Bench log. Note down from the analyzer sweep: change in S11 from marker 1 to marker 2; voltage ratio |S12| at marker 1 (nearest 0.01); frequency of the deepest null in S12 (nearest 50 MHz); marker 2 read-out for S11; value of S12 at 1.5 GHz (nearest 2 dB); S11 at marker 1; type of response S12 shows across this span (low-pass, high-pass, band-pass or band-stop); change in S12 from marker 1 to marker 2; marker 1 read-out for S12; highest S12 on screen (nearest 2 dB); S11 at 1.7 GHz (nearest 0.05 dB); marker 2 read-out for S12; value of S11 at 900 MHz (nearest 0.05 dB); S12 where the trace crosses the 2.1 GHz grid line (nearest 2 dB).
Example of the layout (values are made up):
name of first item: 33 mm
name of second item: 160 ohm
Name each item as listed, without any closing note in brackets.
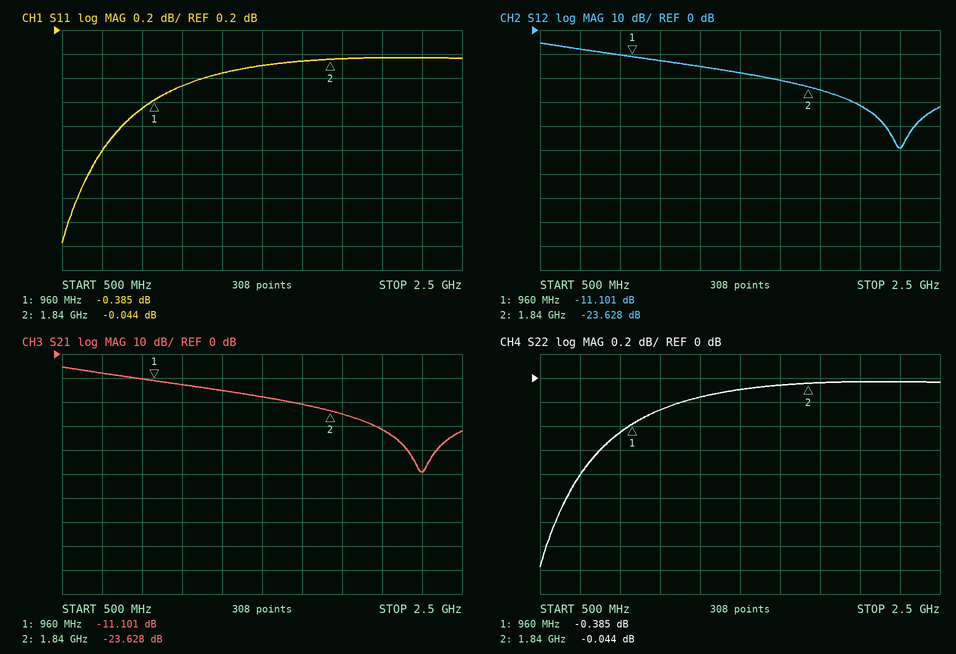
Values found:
change in S11 from marker 1 to marker 2: 0.341 dB
voltage ratio |S12| at marker 1: 0.28
frequency of the deepest null in S12: 2.30 GHz
marker 2 read-out for S11: -0.044 dB
value of S12 at 1.5 GHz: -18 dB
S11 at marker 1: -0.385 dB
type of response S12 shows across this span: low-pass
change in S12 from marker 1 to marker 2: -12.527 dB
marker 1 read-out for S12: -11.101 dB
highest S12 on screen: -6 dB
S11 at 1.7 GHz: -0.05 dB
marker 2 read-out for S12: -23.628 dB
value of S11 at 900 MHz: -0.45 dB
S12 where the trace crosses the 2.1 GHz grid line: -32 dB
